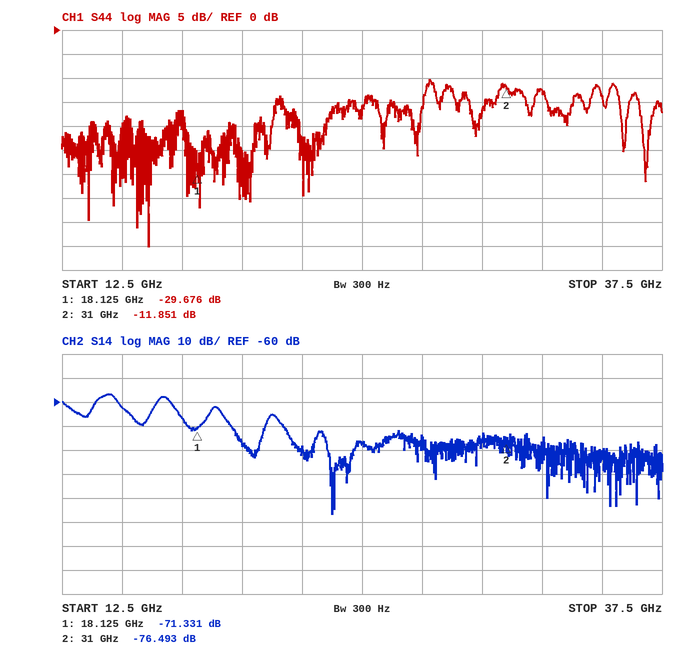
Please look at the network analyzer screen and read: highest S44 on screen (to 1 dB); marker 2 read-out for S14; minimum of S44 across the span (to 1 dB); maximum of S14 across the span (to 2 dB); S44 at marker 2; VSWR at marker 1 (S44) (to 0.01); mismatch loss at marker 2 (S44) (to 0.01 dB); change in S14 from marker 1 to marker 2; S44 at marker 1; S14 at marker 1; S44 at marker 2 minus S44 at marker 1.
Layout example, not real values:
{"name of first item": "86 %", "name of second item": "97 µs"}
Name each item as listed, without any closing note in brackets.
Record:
{"highest S44 on screen": "-10 dB", "marker 2 read-out for S14": "-76.493 dB", "minimum of S44 across the span": "-45 dB", "maximum of S14 across the span": "-56 dB", "S44 at marker 2": "-11.851 dB", "VSWR at marker 1 (S44)": "1.07", "mismatch loss at marker 2 (S44)": "0.29 dB", "change in S14 from marker 1 to marker 2": "-5.162 dB", "S44 at marker 1": "-29.676 dB", "S14 at marker 1": "-71.331 dB", "S44 at marker 2 minus S44 at marker 1": "17.825 dB"}
